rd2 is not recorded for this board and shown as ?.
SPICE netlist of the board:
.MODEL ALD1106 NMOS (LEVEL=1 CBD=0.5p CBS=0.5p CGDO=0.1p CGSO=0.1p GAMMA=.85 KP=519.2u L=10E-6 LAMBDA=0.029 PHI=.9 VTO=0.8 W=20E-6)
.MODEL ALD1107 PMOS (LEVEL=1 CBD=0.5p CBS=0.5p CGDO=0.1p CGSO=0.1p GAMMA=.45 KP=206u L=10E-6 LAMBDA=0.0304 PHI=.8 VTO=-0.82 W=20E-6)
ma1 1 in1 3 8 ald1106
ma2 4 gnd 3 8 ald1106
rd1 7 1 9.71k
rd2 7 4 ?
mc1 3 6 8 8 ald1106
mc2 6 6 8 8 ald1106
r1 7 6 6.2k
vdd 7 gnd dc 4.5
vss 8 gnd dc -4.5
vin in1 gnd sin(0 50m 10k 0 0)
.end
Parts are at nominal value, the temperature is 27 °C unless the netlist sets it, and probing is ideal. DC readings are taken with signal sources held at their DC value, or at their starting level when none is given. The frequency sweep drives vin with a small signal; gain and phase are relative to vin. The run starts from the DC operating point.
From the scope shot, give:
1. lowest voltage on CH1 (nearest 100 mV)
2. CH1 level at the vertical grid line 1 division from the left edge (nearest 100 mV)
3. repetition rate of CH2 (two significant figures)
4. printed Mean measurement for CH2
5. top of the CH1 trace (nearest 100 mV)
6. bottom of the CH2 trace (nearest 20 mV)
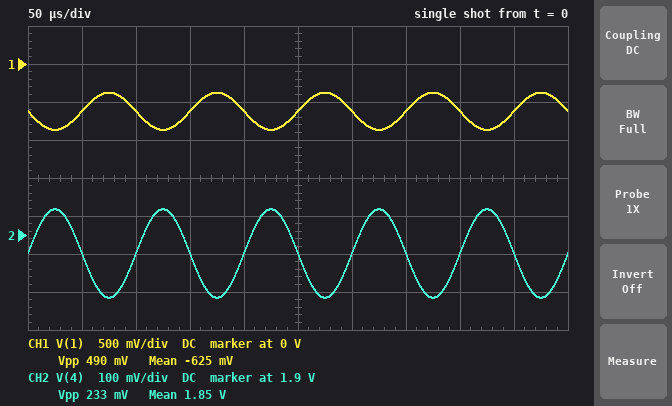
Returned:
-900 mV
-600 mV
10 kHz
1.85 V
-400 mV
1.74 V
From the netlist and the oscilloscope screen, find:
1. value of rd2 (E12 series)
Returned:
4.7 kΩ
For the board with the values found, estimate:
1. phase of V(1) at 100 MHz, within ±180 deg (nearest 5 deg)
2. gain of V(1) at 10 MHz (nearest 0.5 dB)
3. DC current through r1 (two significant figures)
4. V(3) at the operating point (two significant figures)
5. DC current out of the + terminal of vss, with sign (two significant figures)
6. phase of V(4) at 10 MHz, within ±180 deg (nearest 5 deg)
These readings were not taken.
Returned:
140 deg
14.0 dB
1.1 mA
-2.4 V
-2.2 mA
-5 deg
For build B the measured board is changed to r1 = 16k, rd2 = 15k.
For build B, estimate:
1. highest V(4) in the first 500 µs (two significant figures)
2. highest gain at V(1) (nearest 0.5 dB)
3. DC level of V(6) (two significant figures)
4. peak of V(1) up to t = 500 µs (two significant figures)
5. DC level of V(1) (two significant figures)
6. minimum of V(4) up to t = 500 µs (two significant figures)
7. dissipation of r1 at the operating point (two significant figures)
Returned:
1.3 V
10.5 dB
-2.8 V
2.4 V
2.2 V
820 mV
3.3 mW
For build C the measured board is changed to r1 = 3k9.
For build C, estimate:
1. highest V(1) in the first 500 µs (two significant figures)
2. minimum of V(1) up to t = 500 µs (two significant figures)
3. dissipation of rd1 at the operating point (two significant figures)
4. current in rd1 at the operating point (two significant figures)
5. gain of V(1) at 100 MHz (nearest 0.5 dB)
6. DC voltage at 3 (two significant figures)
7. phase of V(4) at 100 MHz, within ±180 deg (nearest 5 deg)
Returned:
-2.0 V
-2.1 V
4.4 mW
670 µA
-3.0 dB
-2.7 V
-5 deg
